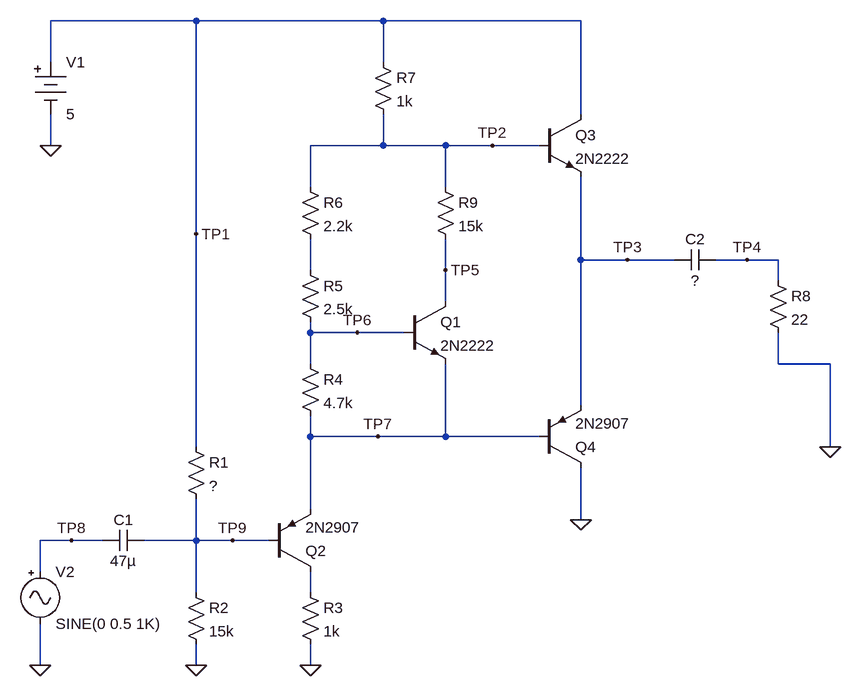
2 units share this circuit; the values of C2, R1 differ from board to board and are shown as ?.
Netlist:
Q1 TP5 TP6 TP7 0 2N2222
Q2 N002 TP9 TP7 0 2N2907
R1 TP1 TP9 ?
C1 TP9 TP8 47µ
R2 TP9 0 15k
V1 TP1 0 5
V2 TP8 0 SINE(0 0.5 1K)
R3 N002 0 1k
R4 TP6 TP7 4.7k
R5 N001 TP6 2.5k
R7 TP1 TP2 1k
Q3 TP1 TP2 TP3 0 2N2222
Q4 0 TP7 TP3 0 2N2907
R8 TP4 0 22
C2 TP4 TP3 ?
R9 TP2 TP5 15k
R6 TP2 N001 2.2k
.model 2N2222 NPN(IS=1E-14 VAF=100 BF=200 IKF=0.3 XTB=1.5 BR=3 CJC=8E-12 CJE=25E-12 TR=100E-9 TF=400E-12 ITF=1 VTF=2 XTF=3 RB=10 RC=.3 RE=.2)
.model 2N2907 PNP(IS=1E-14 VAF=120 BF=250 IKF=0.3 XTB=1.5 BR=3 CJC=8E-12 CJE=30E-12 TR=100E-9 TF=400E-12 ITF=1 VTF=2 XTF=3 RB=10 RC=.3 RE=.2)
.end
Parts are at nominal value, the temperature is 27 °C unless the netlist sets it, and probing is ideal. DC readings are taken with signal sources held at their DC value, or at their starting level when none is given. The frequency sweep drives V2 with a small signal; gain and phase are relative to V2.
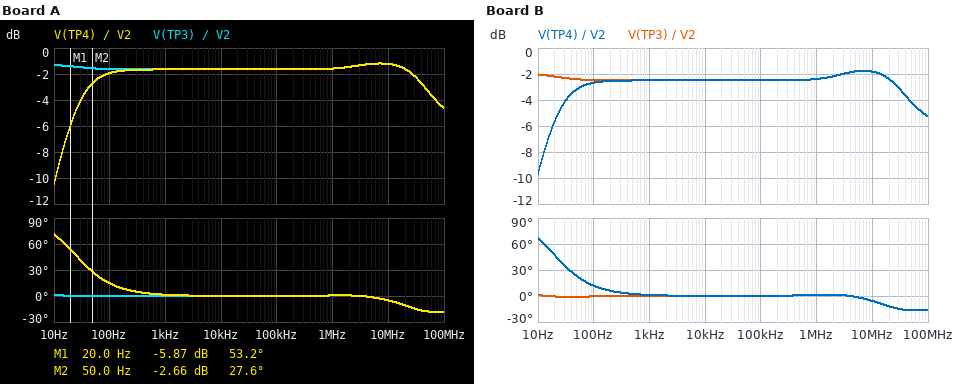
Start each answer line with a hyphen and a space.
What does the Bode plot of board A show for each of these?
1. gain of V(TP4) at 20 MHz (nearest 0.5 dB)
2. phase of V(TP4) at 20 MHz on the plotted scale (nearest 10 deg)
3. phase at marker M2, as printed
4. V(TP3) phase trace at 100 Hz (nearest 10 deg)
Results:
- -1.5 dB
- -10 deg
- 27.6 deg
- 0 deg
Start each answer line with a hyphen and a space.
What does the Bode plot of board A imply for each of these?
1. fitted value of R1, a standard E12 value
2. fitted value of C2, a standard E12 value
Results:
- 18 kΩ
- 270 µF
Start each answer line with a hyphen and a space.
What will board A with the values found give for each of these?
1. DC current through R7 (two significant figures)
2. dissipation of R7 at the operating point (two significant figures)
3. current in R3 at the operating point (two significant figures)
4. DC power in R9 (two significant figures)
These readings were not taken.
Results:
- 540 µA
- 290 µW
- 490 µA
- 150 µW
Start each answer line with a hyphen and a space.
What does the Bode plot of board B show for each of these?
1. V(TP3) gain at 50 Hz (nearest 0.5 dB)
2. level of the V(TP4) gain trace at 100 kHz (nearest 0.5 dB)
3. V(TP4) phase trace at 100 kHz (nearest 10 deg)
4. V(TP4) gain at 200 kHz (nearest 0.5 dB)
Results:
- -2.5 dB
- -2.5 dB
- 0 deg
- -2.5 dB
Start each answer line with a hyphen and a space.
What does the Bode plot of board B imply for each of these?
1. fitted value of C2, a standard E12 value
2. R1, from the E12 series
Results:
- 330 µF
- 15 kΩ
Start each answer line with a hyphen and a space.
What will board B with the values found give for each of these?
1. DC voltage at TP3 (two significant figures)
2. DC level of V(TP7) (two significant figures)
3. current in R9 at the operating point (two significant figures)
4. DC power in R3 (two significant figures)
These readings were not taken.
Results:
- 3.9 V
- 3.1 V
- 97 µA
- 130 µW
